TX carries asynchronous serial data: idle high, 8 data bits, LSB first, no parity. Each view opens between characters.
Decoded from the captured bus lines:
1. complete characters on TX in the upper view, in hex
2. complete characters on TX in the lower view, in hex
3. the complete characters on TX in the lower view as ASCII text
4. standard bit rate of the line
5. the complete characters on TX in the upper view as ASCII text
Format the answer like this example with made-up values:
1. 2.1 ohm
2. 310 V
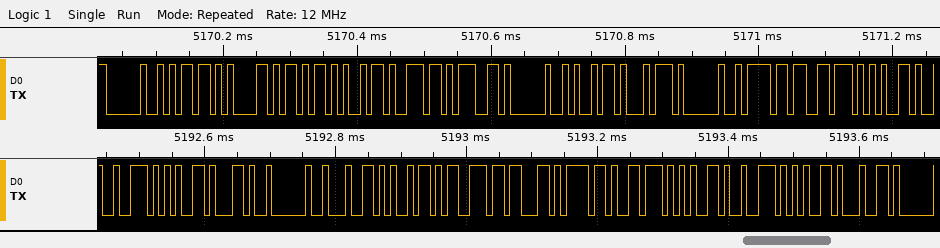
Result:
1. 20, 6D, 61, 6B, 69, 6E, 67, 20, 69, 74, 20, 6F, 76, 65
2. 72, 65, 2C, 20, 64, 69, 73, 63, 6F, 76, 65, 72, 65, 64
3. "re, discovered"
4. 115200 baud
5. " making it ove"
